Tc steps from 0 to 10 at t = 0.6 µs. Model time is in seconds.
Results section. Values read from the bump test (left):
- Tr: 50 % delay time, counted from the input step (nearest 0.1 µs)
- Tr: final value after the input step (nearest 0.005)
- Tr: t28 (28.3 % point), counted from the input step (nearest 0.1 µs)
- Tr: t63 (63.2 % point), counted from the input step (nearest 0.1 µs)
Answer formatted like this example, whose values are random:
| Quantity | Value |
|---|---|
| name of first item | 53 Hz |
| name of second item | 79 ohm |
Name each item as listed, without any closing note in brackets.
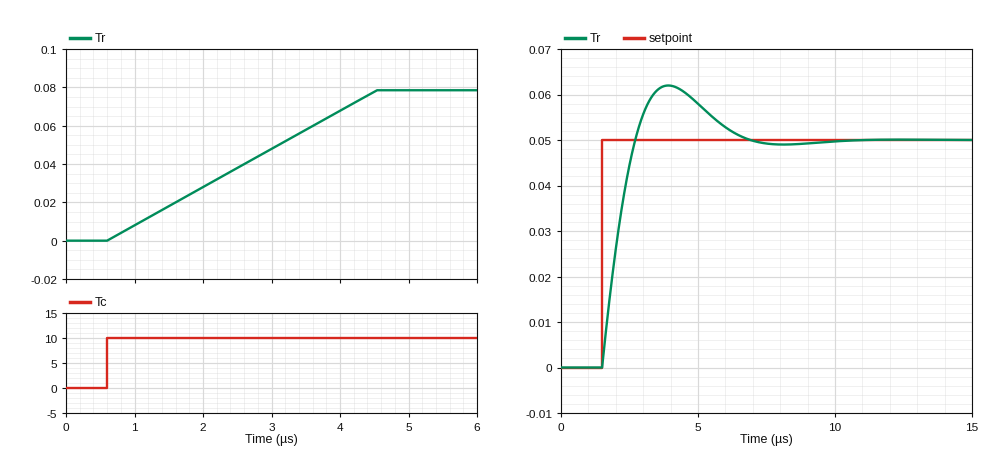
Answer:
| Quantity | Value |
|---|---|
| Tr: 50 % delay time, counted from the input step | 2.0 µs |
| Tr: final value after the input step | 0.080 |
| Tr: t28 (28.3 % point), counted from the input step | 1.1 µs |
| Tr: t63 (63.2 % point), counted from the input step | 2.5 µs |
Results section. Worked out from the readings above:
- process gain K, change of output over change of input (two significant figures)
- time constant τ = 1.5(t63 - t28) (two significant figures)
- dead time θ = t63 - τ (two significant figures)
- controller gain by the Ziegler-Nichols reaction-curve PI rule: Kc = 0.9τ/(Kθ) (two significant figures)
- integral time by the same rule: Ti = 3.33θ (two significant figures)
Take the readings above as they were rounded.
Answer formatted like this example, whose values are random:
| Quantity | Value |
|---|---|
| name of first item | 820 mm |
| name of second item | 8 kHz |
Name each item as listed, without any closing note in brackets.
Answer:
| Quantity | Value |
|---|---|
| process gain K, change of output over change of input | 0.0080 |
| time constant τ = 1.5(t63 - t28) | 2.1 µs |
| dead time θ = t63 - τ | 0.40 µs |
| controller gain by the Ziegler-Nichols reaction-curve PI rule: Kc = 0.9τ/(Kθ) | 590 |
| integral time by the same rule: Ti = 3.33θ | 1.3 µs |
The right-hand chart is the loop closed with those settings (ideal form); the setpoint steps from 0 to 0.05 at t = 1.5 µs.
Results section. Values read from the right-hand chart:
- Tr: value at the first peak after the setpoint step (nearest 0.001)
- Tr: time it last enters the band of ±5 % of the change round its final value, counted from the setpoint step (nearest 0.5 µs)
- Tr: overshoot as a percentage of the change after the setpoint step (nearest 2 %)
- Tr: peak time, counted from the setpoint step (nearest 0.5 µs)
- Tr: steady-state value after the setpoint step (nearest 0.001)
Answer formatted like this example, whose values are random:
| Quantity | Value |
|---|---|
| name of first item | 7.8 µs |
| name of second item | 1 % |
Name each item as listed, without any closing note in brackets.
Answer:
| Quantity | Value |
|---|---|
| Tr: value at the first peak after the setpoint step | 0.062 |
| Tr: time it last enters the band of ±5 % of the change round its final value, counted from the setpoint step | 4.5 µs |
| Tr: overshoot as a percentage of the change after the setpoint step | 24 % |
| Tr: peak time, counted from the setpoint step | 2.5 µs |
| Tr: steady-state value after the setpoint step | 0.050 |
